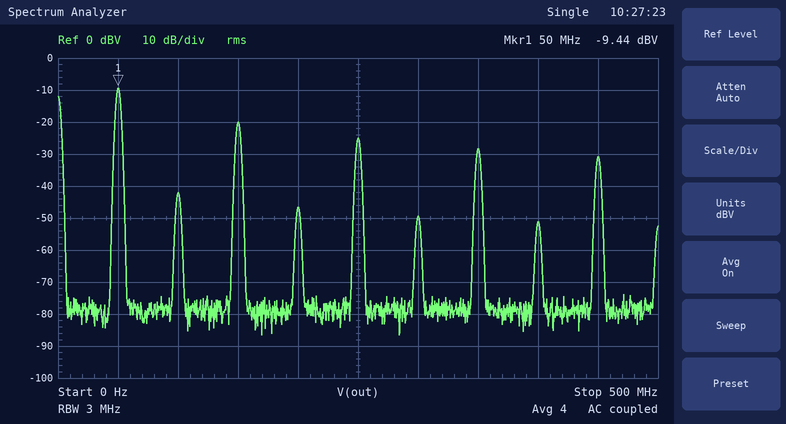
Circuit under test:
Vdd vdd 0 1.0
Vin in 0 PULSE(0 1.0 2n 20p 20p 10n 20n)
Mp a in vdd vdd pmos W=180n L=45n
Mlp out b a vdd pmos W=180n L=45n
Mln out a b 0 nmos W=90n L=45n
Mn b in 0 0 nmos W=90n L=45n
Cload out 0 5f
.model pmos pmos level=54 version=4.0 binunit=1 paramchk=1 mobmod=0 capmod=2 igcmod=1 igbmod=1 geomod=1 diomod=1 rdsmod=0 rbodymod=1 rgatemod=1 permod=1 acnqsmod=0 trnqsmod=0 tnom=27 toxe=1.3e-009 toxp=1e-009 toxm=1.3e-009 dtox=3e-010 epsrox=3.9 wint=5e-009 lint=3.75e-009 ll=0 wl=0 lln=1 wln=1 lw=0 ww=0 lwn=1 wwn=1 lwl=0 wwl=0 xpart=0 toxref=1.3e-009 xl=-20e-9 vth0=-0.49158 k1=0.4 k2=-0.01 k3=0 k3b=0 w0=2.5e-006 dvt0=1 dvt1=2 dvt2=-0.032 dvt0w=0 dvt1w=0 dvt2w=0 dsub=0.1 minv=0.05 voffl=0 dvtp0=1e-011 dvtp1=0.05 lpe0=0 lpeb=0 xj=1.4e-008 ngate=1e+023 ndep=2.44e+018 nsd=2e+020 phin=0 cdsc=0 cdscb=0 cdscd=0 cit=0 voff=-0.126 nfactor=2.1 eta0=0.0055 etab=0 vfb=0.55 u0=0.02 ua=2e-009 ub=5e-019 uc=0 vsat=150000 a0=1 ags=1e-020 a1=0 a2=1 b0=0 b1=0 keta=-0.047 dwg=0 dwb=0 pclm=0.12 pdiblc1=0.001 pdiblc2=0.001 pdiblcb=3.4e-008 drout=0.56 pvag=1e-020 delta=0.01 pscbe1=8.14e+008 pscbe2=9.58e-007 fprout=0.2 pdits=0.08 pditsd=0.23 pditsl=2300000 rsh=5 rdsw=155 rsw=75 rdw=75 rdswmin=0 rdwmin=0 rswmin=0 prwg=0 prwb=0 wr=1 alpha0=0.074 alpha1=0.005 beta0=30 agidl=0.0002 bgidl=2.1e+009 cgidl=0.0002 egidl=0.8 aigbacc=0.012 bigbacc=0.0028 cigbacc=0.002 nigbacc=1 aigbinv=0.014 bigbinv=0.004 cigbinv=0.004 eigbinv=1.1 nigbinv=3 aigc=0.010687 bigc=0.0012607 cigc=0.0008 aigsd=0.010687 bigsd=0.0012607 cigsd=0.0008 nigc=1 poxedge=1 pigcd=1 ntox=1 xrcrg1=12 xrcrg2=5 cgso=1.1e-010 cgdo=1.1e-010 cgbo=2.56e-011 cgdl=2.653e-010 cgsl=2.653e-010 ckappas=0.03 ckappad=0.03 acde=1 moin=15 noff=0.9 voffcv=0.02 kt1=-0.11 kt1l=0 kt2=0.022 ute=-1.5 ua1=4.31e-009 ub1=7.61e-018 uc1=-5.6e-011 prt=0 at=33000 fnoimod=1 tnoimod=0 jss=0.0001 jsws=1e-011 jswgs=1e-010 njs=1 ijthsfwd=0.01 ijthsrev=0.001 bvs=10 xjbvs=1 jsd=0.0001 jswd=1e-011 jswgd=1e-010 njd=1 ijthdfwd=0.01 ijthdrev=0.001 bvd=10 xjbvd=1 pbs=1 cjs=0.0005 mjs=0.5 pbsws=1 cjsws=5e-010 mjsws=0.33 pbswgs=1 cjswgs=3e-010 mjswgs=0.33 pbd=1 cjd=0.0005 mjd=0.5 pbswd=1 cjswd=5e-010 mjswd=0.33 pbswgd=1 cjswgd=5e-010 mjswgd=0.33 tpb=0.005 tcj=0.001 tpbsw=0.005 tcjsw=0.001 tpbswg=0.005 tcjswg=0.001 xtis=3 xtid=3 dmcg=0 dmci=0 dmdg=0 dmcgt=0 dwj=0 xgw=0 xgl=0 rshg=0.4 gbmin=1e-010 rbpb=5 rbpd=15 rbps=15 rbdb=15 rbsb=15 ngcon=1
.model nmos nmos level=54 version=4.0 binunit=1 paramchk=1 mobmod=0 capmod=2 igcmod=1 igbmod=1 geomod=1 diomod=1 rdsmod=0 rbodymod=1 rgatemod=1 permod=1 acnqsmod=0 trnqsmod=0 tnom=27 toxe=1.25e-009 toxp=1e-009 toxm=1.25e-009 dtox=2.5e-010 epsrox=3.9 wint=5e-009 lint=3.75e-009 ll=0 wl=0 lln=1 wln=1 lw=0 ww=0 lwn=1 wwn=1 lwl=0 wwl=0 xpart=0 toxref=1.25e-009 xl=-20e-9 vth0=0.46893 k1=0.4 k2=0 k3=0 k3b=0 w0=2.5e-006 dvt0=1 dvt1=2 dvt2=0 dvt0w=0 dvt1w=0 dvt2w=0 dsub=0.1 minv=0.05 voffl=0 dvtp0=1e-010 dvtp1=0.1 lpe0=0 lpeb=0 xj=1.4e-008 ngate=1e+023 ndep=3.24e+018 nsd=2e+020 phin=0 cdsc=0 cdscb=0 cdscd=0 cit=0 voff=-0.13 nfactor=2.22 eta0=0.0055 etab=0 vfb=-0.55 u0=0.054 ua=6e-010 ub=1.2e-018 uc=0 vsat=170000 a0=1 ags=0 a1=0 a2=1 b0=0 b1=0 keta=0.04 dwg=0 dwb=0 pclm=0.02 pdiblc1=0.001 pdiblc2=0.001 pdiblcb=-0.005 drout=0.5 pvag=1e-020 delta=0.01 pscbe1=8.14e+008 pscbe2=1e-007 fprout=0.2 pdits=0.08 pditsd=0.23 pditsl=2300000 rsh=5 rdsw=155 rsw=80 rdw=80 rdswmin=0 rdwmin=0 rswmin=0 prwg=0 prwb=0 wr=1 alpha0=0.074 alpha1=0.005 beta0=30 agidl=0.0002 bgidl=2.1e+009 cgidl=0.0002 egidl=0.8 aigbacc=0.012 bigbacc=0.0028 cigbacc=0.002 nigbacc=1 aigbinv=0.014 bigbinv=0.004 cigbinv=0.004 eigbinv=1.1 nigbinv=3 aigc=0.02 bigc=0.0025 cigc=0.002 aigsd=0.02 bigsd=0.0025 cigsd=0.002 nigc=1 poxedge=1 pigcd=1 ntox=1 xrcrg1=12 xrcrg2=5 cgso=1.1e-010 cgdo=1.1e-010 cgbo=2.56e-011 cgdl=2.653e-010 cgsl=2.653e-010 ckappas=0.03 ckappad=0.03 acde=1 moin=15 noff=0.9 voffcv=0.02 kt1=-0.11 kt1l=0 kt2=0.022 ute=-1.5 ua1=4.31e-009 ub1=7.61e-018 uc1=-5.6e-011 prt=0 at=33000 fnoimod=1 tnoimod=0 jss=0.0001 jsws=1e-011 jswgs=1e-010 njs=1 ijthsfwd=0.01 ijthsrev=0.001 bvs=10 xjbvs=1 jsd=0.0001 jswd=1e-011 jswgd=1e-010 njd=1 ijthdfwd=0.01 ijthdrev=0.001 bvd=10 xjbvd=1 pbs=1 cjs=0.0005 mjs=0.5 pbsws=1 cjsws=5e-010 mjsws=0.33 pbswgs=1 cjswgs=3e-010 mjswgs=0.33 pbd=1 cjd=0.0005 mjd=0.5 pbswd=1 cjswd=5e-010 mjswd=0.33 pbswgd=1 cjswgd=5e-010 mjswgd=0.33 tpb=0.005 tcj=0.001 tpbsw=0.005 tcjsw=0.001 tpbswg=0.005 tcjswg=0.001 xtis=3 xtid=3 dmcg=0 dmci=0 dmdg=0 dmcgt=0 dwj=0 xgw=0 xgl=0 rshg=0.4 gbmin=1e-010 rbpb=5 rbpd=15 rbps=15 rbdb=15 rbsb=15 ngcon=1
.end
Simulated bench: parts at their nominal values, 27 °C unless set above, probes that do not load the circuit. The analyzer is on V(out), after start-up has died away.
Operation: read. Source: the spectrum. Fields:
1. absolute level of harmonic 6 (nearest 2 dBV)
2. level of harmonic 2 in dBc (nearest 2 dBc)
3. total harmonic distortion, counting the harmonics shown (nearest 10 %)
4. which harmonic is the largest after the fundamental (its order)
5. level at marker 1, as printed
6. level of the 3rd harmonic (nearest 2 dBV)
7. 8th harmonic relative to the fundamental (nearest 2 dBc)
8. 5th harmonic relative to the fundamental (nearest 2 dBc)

-50 dBV
-32 dBc
40 %
3
-9.44 dBV
-20 dBV
-42 dBc
-16 dBc
